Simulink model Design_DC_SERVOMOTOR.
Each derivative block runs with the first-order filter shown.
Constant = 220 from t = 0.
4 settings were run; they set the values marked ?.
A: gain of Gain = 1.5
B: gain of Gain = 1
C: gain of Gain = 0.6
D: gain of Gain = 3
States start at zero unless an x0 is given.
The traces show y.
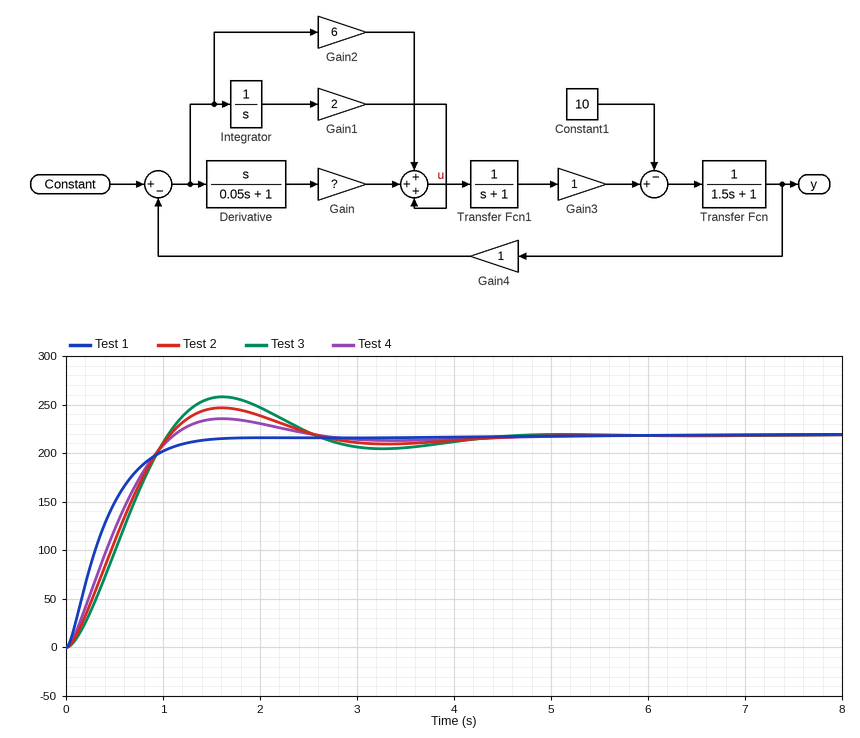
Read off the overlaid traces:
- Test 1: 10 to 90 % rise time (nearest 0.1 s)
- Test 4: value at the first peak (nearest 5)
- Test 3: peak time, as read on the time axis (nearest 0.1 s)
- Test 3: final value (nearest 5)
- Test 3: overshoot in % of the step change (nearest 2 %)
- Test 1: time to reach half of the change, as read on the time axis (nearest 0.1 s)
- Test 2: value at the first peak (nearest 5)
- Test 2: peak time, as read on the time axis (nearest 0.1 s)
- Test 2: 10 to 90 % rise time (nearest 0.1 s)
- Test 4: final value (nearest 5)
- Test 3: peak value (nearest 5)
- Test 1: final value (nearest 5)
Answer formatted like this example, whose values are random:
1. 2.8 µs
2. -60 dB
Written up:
1. 0.8 s
2. 235
3. 1.6 s
4. 220
5. 18 %
6. 0.3 s
7. 245
8. 1.6 s
9. 0.8 s
10. 220
11. 260
12. 220
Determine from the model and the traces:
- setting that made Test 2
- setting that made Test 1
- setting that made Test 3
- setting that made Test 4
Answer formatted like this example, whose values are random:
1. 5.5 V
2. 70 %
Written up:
1. B
2. D
3. C
4. A
